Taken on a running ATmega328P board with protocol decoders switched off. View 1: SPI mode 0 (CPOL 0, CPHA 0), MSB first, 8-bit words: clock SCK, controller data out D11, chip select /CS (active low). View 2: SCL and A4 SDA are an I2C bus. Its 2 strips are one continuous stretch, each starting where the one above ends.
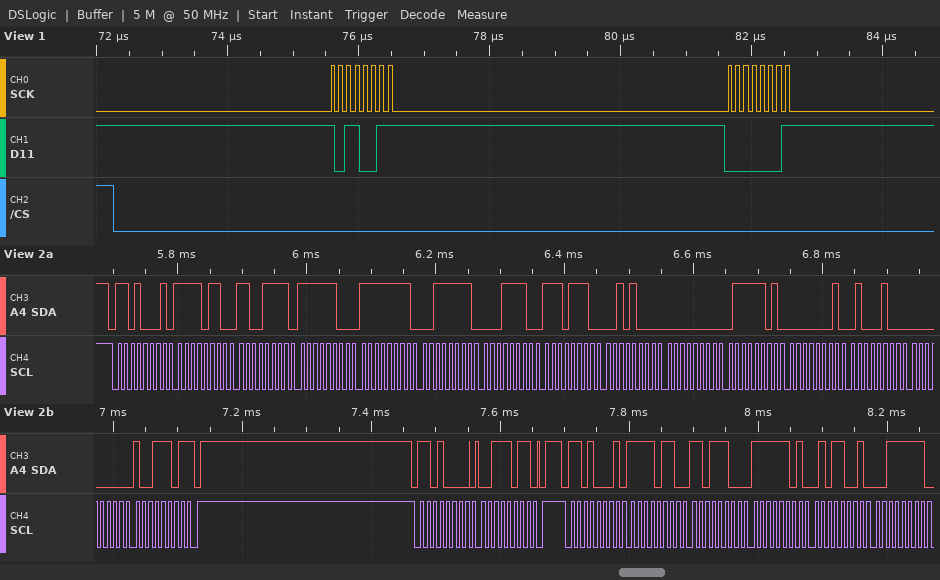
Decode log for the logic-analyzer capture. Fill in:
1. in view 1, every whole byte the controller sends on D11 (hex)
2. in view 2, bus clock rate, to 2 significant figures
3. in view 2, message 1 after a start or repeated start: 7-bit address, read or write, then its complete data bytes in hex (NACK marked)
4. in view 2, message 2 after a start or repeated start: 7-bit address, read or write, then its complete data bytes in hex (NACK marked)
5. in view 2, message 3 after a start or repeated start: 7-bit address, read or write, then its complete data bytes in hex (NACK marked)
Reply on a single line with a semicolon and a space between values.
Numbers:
0xB3 0x01; 100 kHz; 0x68 read: F6 CF FC FF 3F 1E EE 28 00 7D 01 44 00 9D NACK; 0x68 write: 3B; 0x68 read: F6 DC FD 59 3F
